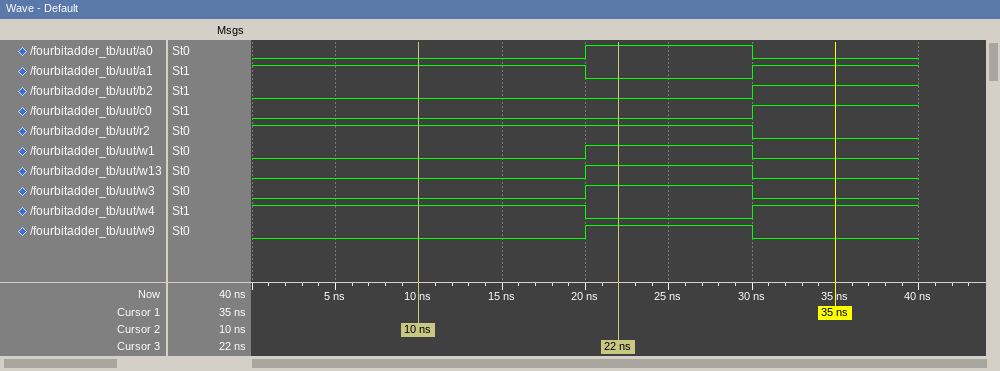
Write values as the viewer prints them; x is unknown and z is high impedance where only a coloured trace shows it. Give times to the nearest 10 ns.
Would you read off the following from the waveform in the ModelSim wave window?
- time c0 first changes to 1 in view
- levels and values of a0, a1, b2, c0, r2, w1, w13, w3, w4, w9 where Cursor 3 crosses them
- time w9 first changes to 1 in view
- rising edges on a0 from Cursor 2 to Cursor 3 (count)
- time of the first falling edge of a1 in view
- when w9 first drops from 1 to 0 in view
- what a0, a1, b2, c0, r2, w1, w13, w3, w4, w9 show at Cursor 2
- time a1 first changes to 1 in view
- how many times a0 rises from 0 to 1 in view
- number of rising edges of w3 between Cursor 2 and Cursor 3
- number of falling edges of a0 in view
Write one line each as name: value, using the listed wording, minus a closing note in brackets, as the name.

time c0 first changes to 1 in view: 30 ns
levels and values of a0, a1, b2, c0, r2, w1, w13, w3, w4, w9 where Cursor 3 crosses them: a0=1, a1=0, b2=0, c0=0, r2=1, w1=1, w13=1, w3=1, w4=0, w9=1
time w9 first changes to 1 in view: 20 ns
rising edges on a0 from Cursor 2 to Cursor 3: 1
time of the first falling edge of a1 in view: 20 ns
when w9 first drops from 1 to 0 in view: 30 ns
what a0, a1, b2, c0, r2, w1, w13, w3, w4, w9 show at Cursor 2: a0=0, a1=1, b2=0, c0=0, r2=1, w1=0, w13=0, w3=0, w4=1, w9=0
time a1 first changes to 1 in view: 30 ns
how many times a0 rises from 0 to 1 in view: 1
number of rising edges of w3 between Cursor 2 and Cursor 3: 1
number of falling edges of a0 in view: 1
